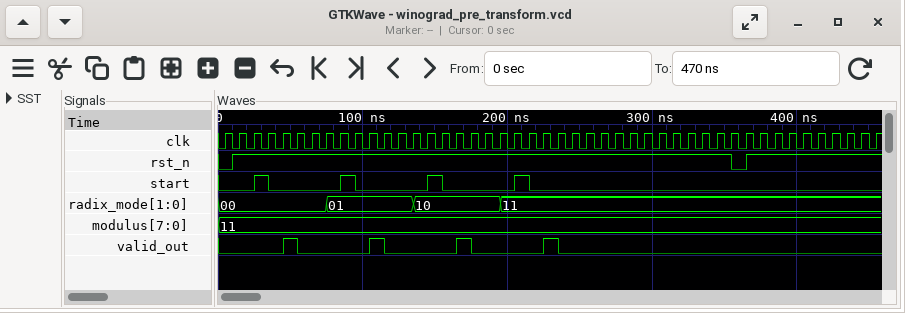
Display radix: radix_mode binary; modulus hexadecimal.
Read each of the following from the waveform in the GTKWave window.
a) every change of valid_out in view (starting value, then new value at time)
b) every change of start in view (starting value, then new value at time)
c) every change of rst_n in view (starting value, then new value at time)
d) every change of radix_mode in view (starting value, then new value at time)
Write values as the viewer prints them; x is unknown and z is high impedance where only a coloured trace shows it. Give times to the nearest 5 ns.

0, 1 at 45 ns, 0 at 55 ns, 1 at 105 ns, 0 at 115 ns, 1 at 165 ns, 0 at 175 ns, 1 at 225 ns, 0 at 235 ns
0, 1 at 25 ns, 0 at 35 ns, 1 at 85 ns, 0 at 95 ns, 1 at 145 ns, 0 at 155 ns, 1 at 205 ns, 0 at 215 ns
0, 1 at 10 ns, 0 at 355 ns, 1 at 365 ns
00, 01 at 75 ns, 10 at 135 ns, 11 at 195 ns
